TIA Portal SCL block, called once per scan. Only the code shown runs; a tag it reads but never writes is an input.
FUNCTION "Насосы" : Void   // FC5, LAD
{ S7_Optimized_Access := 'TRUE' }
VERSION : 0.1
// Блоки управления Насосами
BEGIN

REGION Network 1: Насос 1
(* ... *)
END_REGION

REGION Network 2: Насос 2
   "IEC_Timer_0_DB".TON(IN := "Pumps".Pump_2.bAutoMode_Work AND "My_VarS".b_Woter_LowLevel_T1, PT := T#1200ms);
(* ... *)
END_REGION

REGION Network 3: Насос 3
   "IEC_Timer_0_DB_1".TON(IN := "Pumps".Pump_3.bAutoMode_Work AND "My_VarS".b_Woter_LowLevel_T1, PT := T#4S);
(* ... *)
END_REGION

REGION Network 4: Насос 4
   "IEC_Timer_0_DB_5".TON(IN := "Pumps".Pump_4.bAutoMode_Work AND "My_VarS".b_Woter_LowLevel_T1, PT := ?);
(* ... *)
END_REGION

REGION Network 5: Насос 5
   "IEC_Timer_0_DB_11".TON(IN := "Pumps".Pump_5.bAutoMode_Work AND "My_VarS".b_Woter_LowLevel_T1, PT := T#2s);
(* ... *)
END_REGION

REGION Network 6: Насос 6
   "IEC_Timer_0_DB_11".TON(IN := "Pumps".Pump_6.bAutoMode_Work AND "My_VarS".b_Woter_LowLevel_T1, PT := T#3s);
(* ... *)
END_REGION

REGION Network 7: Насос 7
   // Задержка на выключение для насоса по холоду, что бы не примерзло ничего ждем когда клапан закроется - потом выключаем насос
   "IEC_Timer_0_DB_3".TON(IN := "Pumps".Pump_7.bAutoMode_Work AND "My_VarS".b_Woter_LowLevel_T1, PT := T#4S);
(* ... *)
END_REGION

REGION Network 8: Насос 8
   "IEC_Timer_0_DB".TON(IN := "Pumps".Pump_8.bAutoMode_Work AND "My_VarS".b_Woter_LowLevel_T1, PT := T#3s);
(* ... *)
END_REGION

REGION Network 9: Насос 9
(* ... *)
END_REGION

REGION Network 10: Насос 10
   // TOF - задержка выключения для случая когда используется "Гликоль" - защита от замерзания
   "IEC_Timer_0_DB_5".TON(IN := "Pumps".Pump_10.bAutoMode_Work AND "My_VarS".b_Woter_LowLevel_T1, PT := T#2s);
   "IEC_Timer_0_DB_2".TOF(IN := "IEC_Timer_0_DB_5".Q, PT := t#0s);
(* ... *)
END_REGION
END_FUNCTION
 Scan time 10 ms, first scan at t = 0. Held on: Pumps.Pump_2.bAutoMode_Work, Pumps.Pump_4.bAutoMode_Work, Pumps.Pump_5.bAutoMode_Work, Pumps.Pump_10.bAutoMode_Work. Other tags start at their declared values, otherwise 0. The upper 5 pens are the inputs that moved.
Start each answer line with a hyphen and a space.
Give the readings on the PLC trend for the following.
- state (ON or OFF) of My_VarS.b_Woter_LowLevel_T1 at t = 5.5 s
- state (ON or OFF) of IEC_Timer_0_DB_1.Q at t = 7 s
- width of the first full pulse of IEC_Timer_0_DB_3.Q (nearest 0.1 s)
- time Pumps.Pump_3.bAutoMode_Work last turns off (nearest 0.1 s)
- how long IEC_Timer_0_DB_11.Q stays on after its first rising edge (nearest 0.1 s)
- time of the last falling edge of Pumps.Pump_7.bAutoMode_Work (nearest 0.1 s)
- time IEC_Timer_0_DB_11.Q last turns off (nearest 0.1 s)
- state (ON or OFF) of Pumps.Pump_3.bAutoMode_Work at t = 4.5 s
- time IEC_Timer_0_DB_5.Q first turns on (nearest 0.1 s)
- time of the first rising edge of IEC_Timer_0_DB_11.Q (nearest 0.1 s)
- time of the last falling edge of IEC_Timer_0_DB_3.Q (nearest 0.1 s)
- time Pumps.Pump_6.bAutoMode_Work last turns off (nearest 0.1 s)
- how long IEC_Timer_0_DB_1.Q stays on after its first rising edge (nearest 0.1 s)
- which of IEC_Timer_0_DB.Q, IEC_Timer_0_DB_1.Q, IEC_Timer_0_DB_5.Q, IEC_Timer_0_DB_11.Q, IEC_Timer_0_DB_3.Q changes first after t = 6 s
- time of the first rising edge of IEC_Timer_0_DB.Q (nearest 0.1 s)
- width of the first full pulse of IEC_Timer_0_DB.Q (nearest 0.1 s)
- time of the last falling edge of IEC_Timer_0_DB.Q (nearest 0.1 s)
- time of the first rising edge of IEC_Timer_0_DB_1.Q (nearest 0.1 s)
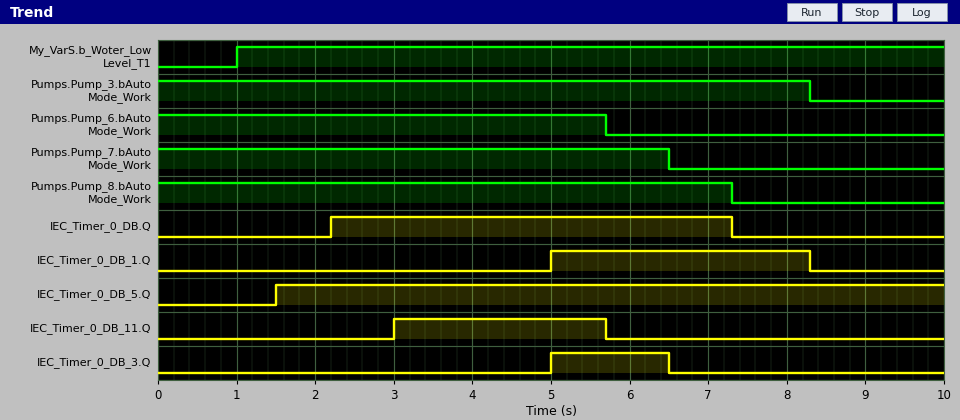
- ON
- ON
- 1.5 s
- 8.3 s
- 2.7 s
- 6.5 s
- 5.7 s
- ON
- 1.5 s
- 3.0 s
- 6.5 s
- 5.7 s
- 3.3 s
- IEC_Timer_0_DB_3.Q
- 2.2 s
- 5.1 s
- 7.3 s
- 5.0 s
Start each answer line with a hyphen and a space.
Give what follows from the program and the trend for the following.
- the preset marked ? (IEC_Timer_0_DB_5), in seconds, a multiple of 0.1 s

- 0.5 s
